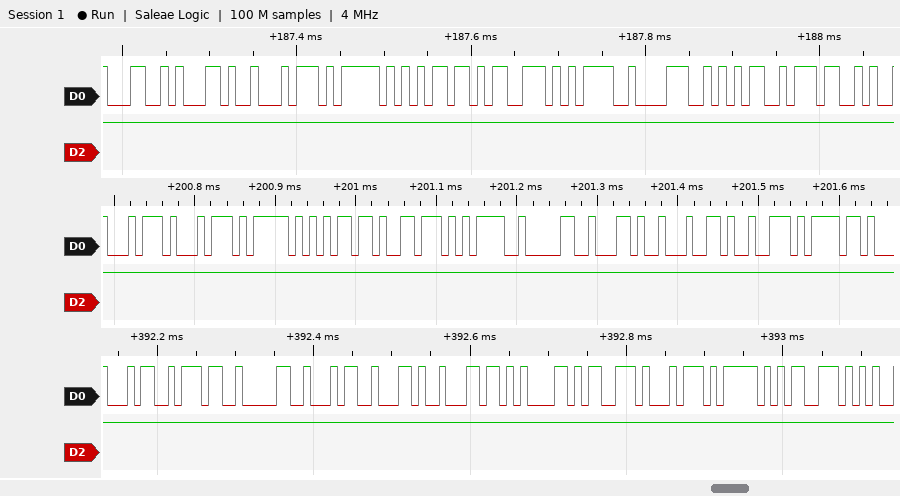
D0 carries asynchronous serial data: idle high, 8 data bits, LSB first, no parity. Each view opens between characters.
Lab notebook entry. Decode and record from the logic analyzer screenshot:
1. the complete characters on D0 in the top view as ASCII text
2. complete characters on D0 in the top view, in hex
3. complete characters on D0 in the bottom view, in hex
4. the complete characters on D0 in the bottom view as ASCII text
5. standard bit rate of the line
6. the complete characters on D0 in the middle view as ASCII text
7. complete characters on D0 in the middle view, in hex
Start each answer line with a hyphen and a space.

- "L,t_ms=857"
- 4C, 2C, 74, 5F, 6D, 73, 3D, 38, 35, 37
- 34, 37, 30, 34, 2C, 6C, 61, 73, 74, 5F, 73
- "4704,last_s"
- 115200 baud
- "tt_mv=0,dro"
- 74, 74, 5F, 6D, 76, 3D, 30, 2C, 64, 72, 6F
